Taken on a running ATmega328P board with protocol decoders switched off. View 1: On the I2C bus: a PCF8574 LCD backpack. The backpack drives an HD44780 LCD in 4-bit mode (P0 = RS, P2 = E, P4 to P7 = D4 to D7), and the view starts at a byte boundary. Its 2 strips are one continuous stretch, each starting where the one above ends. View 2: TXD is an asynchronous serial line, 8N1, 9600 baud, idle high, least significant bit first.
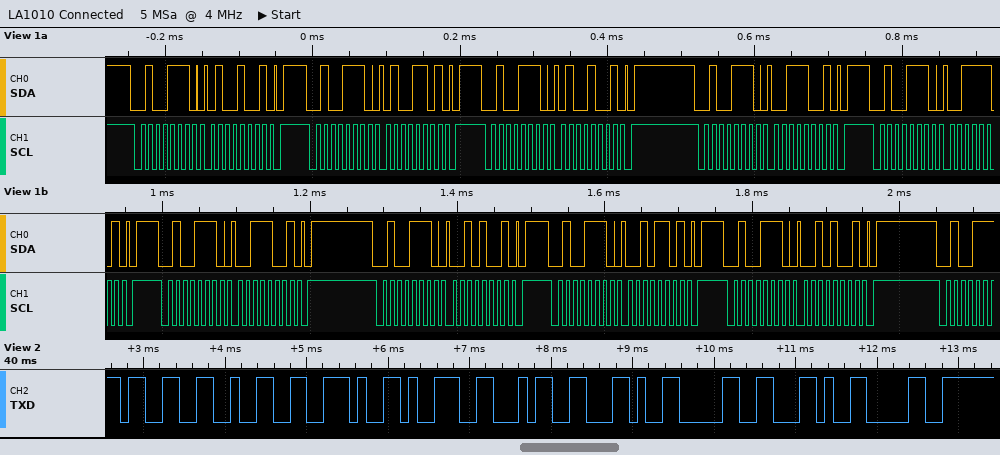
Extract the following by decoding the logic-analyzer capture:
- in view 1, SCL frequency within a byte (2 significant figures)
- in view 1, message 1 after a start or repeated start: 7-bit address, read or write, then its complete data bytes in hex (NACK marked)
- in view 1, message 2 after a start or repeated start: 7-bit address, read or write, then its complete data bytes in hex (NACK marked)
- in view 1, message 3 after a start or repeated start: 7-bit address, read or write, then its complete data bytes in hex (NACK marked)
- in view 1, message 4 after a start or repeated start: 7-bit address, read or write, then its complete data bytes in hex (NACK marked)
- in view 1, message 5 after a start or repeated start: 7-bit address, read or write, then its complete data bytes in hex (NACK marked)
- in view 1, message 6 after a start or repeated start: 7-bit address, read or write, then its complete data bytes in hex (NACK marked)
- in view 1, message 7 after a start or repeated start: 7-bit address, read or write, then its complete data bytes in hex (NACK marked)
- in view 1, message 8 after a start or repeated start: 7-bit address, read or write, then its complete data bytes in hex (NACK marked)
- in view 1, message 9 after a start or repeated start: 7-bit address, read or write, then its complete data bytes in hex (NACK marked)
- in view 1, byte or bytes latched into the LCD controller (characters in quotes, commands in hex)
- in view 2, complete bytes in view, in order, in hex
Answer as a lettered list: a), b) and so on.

a) 100 kHz
b) 0x27 write: 49
c) 0x27 write: 4D
d) 0x27 write: 49
e) 0x27 write: 39
f) 0x27 write: 3D
g) 0x27 write: 39
h) 0x27 write: 29
i) 0x27 write: 2D
j) 0x27 write: 29
k) 'C'
l) 0x33 0x32 0x2E 0x39 0x34 0x2C 0x30 0x2C 0x30
